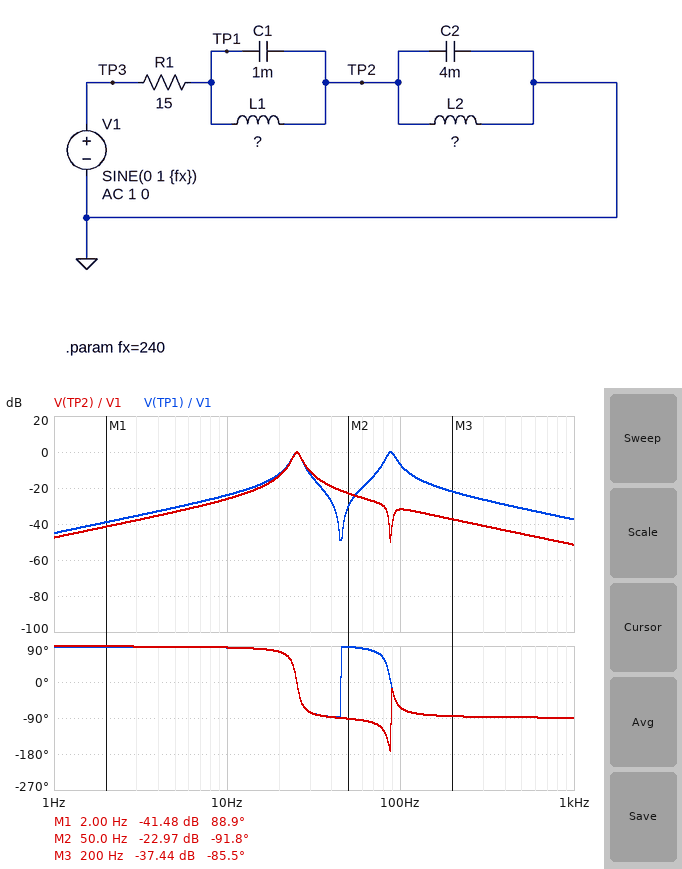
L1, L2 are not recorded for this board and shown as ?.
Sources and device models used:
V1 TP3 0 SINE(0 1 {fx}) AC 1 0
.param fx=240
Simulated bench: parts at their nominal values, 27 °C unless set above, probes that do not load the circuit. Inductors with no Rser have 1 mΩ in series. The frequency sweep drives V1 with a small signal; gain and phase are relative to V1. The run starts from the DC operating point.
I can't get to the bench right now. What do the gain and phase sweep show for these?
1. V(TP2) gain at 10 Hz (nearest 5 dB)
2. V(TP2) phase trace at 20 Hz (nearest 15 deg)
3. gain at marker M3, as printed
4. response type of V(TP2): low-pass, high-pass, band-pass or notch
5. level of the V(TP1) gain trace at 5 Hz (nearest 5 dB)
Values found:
-25 dB
75 deg
-37.44 dB
band-pass
-30 dB
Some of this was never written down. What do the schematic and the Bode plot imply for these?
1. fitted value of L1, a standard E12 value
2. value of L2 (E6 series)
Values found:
3.3 mH
10 mH
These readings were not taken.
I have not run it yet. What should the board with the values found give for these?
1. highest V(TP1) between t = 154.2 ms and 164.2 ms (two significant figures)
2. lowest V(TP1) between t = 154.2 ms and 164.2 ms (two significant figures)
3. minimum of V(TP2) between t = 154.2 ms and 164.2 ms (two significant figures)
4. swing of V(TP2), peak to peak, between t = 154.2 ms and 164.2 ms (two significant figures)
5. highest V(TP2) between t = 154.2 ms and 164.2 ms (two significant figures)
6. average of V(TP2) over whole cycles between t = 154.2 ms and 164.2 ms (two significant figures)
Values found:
65 mV
-60 mV
-8.8 mV
23 mV
14 mV
2.7 mV
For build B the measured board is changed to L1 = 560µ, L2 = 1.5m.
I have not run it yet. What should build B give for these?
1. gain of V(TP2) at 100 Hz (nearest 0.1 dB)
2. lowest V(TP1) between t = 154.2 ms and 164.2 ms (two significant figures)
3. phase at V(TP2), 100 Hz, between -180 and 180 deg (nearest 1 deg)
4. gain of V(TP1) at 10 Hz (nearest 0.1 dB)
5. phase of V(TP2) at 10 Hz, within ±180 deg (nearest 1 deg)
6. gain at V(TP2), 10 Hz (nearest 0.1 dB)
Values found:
-26.8 dB
-220 mV
-89 deg
-41.1 dB
89 deg
-43.8 dB
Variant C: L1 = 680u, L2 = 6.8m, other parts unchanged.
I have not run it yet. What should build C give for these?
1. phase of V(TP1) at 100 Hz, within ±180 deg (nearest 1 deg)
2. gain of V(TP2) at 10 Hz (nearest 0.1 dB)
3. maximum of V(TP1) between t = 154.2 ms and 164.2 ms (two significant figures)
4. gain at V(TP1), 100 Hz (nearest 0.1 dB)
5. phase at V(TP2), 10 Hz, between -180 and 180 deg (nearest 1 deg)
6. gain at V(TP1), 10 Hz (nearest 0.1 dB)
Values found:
89 deg
-29.9 dB
140 mV
-40.3 dB
88 deg
-29.2 dB
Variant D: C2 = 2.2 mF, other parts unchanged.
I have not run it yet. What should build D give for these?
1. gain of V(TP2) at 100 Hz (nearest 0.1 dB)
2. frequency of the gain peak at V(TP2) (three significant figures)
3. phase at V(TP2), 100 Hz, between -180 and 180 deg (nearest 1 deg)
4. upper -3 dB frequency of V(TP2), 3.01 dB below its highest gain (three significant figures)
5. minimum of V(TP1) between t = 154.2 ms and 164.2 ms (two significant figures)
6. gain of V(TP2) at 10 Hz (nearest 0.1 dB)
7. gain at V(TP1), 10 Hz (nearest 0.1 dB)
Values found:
-26.3 dB
34.1 Hz
-63 deg
36.6 Hz
-73 mV
-26.8 dB
-24.5 dB
